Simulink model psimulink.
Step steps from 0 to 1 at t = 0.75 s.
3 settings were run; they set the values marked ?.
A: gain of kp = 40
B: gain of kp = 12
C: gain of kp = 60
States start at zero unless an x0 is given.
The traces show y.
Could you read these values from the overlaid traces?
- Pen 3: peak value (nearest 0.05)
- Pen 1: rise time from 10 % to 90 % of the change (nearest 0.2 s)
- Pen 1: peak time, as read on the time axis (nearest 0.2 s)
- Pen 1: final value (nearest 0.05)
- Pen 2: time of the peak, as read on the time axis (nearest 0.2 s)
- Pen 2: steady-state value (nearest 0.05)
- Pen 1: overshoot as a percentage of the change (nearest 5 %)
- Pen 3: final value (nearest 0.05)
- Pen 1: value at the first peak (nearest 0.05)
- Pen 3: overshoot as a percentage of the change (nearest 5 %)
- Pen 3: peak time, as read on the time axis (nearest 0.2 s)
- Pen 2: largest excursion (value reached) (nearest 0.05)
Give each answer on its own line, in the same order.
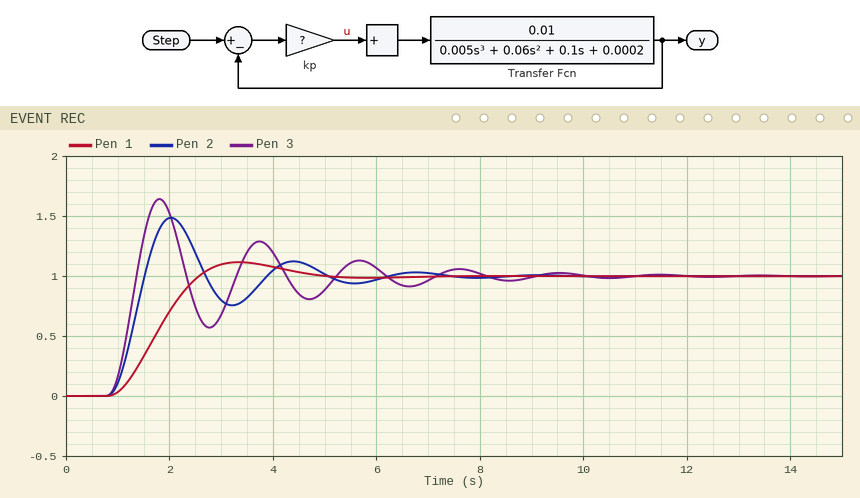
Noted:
1.65
1.2 s
3.4 s
1.00
2.0 s
1.00
10 %
1.00
1.10
65 %
1.8 s
1.50
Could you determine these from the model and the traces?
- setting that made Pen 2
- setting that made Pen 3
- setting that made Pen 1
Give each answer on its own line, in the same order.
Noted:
A
C
B
